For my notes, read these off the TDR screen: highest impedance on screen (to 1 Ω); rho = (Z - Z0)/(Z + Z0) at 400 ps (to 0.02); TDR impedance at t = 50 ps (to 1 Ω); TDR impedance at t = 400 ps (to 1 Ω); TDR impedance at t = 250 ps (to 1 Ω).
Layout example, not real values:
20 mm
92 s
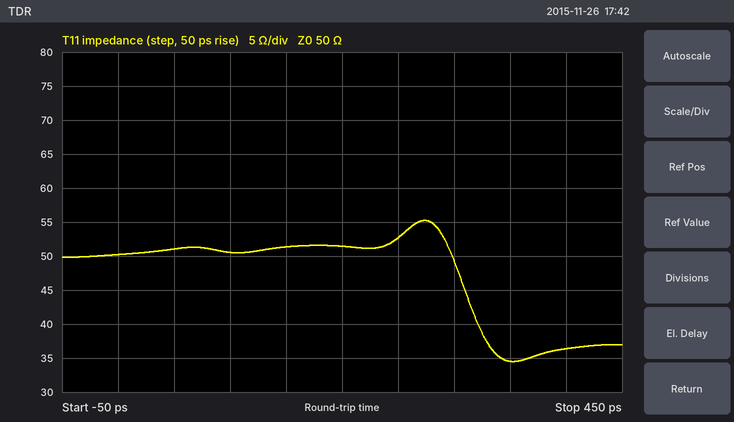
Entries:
55 Ω
-0.16
51 Ω
36 Ω
53 Ω
